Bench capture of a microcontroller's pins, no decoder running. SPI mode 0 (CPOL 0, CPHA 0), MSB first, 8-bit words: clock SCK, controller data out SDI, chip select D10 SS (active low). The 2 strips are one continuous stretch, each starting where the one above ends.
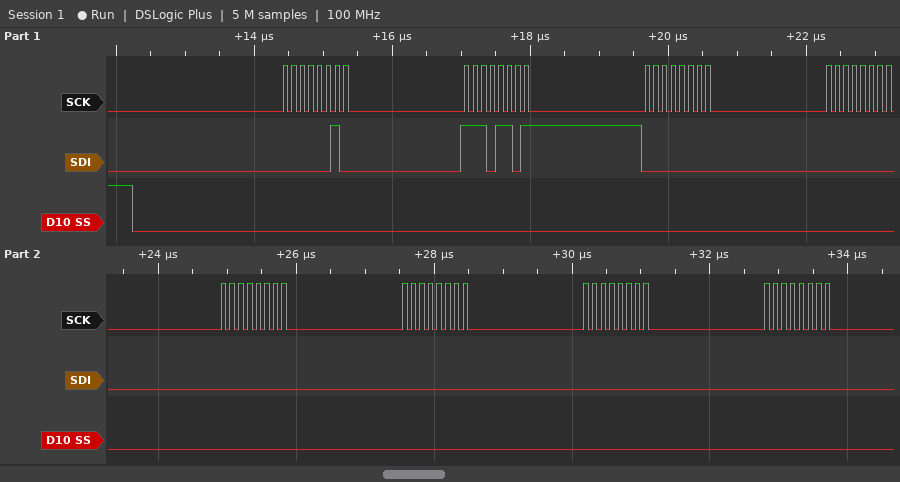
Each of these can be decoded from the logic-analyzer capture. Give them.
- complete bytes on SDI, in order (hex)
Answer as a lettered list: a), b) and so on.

a) 0x02 0xED 0x00 0x00 0x00 0x00 0x00 0x00
